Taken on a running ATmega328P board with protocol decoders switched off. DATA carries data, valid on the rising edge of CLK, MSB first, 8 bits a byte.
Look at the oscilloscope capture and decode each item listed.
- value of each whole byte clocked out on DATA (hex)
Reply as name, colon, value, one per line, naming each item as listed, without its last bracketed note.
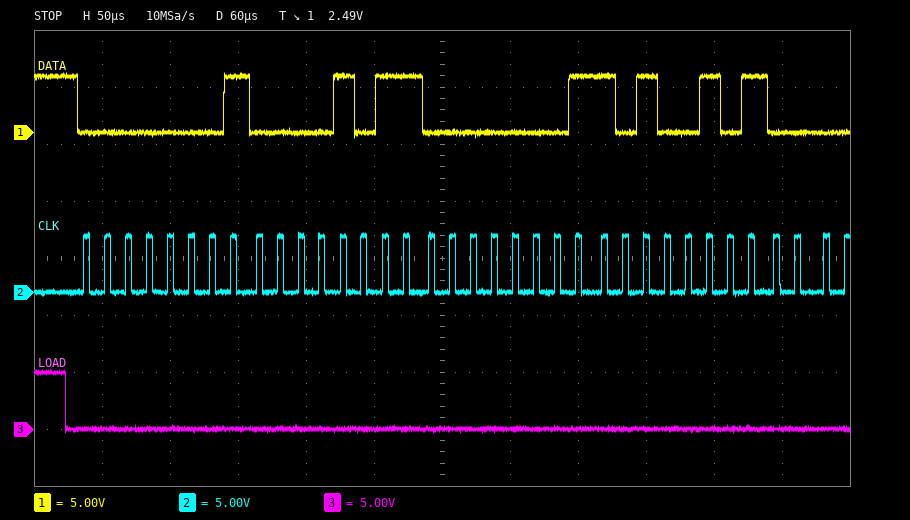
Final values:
value of each whole byte clocked out on DATA: 01 0B 01 A5
